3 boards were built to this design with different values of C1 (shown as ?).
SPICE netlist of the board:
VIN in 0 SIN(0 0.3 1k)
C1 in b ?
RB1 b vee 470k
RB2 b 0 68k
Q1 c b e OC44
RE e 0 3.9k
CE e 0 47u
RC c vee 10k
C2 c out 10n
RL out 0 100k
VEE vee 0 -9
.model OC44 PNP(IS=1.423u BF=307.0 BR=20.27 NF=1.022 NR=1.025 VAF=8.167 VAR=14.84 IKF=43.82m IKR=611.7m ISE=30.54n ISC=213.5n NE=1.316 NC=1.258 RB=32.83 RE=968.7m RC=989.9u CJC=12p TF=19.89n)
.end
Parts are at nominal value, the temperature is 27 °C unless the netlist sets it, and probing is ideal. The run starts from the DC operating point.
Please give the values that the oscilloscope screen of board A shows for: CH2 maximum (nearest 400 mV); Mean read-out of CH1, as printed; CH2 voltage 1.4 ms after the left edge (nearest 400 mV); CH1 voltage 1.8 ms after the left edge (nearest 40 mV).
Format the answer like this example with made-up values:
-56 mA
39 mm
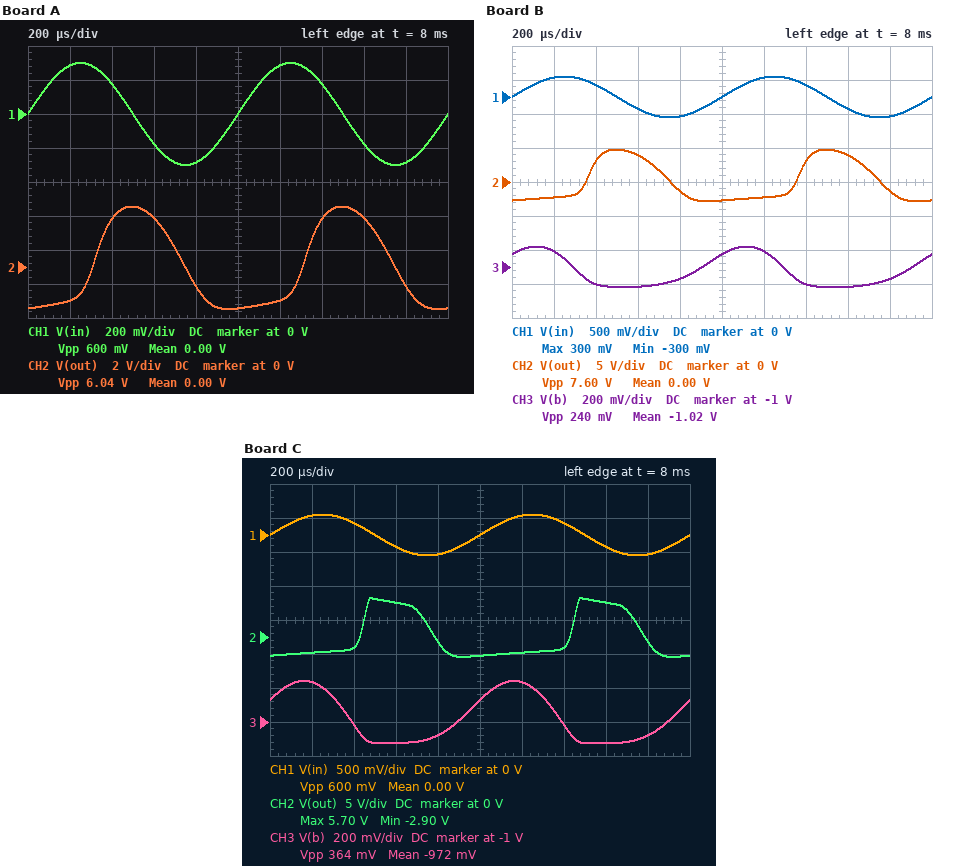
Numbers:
3.6 V
0.00 V
2.8 V
-280 mV
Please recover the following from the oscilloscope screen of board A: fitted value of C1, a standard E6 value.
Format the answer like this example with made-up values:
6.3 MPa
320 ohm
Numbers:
2.2 nF
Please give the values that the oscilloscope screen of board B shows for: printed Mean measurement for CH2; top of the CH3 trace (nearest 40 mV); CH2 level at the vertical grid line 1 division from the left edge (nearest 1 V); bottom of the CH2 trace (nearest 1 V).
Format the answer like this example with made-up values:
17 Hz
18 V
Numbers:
0.00 V
-880 mV
-2 V
-3 V
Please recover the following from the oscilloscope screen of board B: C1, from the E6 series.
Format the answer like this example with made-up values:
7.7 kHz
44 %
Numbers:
3.3 nF
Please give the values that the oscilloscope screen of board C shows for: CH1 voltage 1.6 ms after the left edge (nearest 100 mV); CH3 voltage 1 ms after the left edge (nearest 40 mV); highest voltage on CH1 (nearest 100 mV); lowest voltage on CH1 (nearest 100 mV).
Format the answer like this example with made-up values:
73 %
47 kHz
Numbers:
-200 mV
-880 mV
300 mV
-300 mV
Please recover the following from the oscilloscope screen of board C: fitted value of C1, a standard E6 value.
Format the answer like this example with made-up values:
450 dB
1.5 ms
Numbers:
6.8 nF
